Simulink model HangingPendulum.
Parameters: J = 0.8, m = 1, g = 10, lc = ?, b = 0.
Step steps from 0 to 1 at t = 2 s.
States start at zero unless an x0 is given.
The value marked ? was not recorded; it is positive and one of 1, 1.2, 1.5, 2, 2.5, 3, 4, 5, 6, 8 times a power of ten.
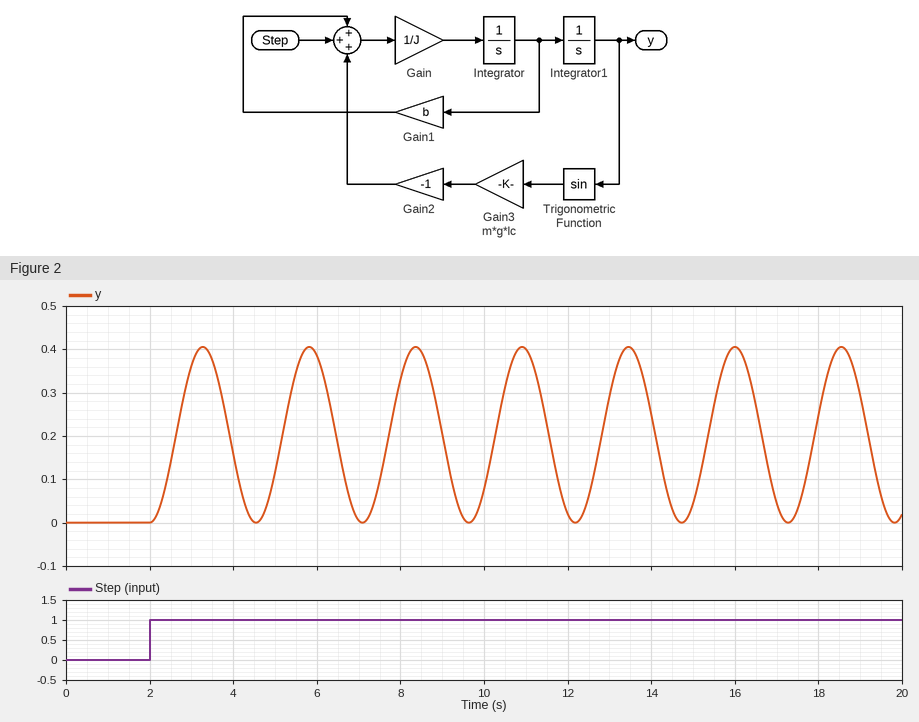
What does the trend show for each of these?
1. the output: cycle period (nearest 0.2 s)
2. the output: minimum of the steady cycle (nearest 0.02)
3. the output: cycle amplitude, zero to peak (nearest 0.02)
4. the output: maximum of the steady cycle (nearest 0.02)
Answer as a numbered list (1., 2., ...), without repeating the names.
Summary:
1. 2.6 s
2. 0.00
3. 0.20
4. 0.40
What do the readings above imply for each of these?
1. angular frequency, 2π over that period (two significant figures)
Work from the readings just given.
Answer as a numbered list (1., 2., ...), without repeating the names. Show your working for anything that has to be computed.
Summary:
1. 2π / 2.6 = 2.4 rad/s
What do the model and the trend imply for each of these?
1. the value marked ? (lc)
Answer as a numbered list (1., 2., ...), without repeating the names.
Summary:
1. 0.5
